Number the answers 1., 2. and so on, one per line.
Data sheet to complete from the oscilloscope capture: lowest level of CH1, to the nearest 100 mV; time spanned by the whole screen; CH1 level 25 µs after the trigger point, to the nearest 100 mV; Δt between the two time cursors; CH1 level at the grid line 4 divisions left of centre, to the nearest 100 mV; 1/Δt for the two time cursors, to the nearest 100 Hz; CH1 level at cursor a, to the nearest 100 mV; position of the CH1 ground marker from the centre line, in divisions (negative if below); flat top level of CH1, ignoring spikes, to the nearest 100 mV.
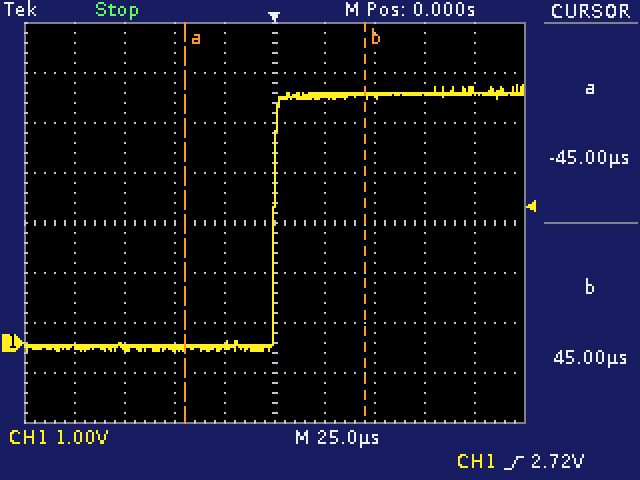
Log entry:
1. -200 mV
2. 250 µs
3. 5.0 V
4. 90.0 µs
5. -100 mV
6. 11.1 kHz
7. -100 mV
8. -2.4 div
9. 5.0 V
